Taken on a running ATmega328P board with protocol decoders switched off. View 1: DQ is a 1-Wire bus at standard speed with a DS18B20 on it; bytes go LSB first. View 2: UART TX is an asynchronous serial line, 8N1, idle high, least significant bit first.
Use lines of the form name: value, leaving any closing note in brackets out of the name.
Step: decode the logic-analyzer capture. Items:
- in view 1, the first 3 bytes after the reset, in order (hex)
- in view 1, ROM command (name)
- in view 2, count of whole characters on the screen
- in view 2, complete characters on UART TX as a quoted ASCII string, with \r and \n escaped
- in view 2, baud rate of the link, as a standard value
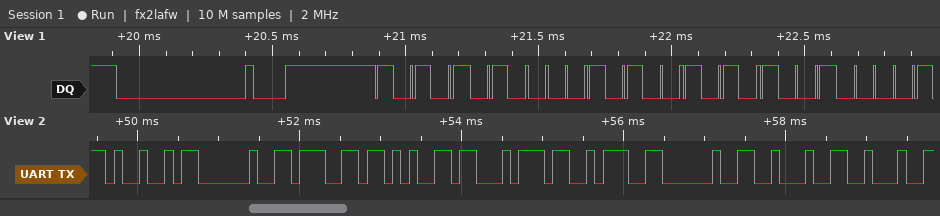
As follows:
in view 1, the first 3 bytes after the reset, in order: 55 28 95
in view 1, ROM command: Match ROM
in view 2, count of whole characters on the screen: 9
in view 2, complete characters on UART TX as a quoted ASCII string, with \r and \n escaped: "I get: \"\""
in view 2, baud rate of the link, as a standard value: 9600 baud
